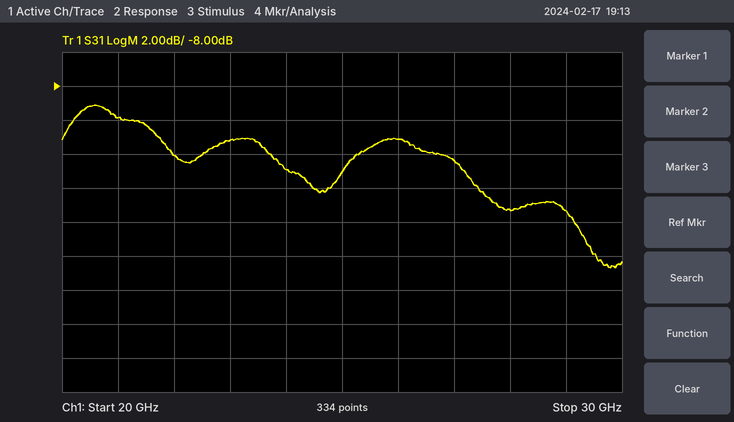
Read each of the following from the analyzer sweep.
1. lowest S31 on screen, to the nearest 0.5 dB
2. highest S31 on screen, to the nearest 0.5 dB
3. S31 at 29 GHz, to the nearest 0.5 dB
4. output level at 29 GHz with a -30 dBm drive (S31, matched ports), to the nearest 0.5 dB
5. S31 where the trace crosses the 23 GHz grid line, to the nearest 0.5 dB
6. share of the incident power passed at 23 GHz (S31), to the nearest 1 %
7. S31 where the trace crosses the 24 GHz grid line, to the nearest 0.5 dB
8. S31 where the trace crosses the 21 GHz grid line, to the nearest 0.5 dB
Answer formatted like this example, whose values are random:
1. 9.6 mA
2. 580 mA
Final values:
1. -18.5 dB
2. -9.0 dB
3. -15.5 dB
4. -45.5 dBm
5. -11.0 dB
6. 8 %
7. -13.0 dB
8. -10.0 dB
